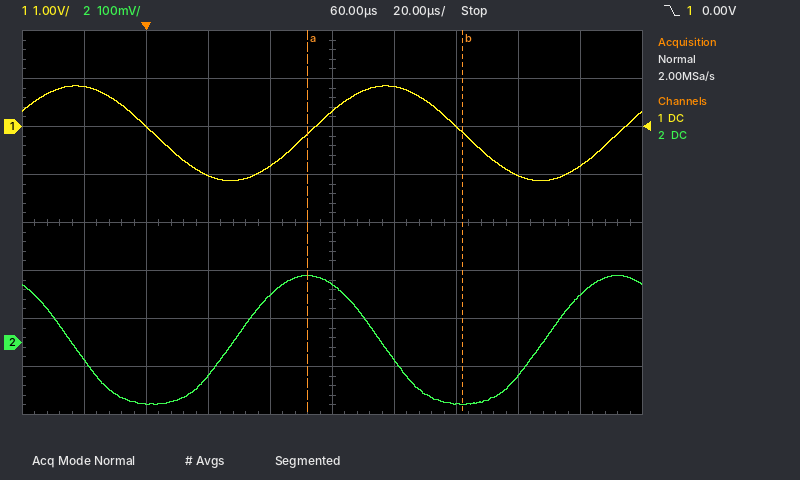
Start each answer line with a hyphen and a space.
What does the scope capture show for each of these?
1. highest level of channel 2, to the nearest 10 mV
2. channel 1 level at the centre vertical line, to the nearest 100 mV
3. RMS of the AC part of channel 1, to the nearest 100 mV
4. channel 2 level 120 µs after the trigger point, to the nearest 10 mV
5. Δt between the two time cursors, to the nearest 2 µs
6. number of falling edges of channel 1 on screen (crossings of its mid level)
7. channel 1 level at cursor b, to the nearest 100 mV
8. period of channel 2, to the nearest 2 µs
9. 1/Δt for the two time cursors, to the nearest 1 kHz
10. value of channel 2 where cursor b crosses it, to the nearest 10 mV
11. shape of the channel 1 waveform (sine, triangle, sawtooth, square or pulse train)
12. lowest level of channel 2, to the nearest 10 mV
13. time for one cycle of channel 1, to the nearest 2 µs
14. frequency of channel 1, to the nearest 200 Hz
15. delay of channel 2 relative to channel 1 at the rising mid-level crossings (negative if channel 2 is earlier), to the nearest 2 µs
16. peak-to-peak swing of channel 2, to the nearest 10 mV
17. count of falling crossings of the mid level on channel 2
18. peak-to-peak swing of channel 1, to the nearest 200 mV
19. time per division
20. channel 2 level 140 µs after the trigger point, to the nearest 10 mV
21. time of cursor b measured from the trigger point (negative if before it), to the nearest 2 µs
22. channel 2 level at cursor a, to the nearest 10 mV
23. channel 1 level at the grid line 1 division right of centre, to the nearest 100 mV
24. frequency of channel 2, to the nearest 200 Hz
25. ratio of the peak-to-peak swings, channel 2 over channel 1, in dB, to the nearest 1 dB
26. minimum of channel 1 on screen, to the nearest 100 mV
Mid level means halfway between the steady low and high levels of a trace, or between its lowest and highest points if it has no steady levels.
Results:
- 140 mV
- 300 mV
- 700 mV
- -70 mV
- 50 µs
- 2
- -100 mV
- 100 µs
- 20 kHz
- -130 mV
- sine
- -130 mV
- 100 µs
- 10.0 kHz
- -24 µs
- 270 mV
- 2
- 2.0 V
- 20 µs
- 100 mV
- +102 µs
- 140 mV
- 800 mV
- 10.0 kHz
- -17 dB
- -1.1 V
